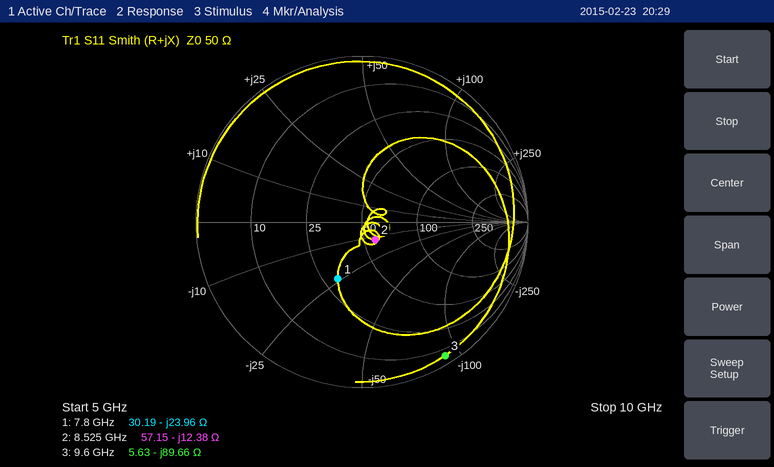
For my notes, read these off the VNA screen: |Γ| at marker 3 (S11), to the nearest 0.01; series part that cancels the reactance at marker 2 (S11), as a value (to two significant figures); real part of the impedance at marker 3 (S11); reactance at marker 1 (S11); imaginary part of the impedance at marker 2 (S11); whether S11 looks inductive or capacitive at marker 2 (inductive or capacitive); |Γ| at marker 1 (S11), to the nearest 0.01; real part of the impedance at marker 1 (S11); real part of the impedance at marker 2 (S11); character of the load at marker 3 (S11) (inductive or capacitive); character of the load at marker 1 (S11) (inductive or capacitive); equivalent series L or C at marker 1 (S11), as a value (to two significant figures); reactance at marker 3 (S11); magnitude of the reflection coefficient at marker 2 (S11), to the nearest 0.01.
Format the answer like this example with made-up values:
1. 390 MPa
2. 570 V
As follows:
1. 0.95
2. 230 pH
3. 5.63 Ω
4. -23.96 Ω
5. -12.38 Ω
6. capacitive
7. 0.37
8. 30.19 Ω
9. 57.15 Ω
10. capacitive
11. capacitive
12. 850 fF
13. -89.66 Ω
14. 0.13
